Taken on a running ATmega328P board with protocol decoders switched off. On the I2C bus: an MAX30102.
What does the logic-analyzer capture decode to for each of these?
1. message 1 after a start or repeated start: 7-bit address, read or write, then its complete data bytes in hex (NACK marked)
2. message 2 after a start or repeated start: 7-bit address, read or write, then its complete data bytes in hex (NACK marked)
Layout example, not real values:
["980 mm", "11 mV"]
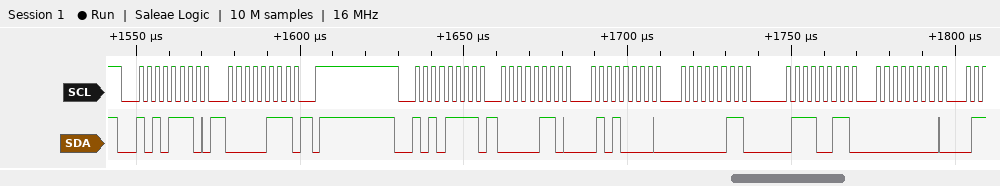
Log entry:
["0x57 write: 07", "0x57 read: 06 50 03 73 00"]
